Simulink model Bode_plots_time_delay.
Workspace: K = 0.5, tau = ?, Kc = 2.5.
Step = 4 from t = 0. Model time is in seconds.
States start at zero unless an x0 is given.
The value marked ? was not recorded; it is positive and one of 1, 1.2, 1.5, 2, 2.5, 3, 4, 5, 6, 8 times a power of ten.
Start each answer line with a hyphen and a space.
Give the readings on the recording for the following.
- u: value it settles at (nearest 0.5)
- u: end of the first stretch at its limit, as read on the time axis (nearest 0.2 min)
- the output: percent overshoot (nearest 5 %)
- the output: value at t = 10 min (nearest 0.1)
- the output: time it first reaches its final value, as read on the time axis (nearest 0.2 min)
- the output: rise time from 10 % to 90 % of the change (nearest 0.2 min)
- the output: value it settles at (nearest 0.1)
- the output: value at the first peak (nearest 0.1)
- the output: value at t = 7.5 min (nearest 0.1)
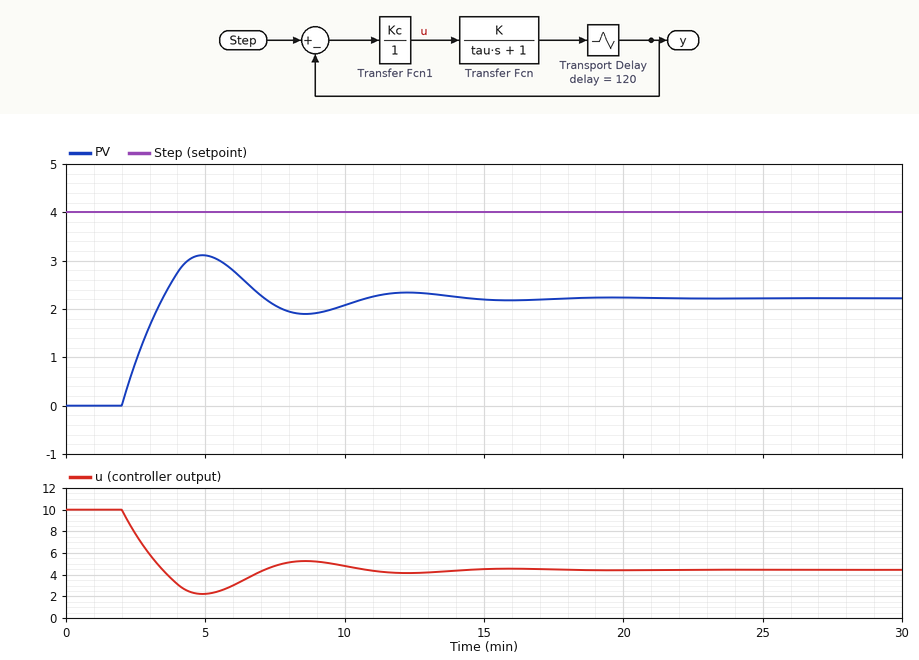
- 4.5
- 2.0 min
- 40 %
- 2.1
- 3.4 min
- 1.2 min
- 2.2
- 3.1
- 2.1
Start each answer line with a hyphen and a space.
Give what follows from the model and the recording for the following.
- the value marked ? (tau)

- 150
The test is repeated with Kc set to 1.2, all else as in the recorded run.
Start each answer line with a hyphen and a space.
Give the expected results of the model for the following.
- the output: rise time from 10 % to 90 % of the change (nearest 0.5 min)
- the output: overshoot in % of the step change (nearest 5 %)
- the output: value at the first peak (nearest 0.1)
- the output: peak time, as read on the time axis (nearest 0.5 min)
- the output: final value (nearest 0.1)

- 2.0 min
- 10 %
- 1.6
- 6.0 min
- 1.5
